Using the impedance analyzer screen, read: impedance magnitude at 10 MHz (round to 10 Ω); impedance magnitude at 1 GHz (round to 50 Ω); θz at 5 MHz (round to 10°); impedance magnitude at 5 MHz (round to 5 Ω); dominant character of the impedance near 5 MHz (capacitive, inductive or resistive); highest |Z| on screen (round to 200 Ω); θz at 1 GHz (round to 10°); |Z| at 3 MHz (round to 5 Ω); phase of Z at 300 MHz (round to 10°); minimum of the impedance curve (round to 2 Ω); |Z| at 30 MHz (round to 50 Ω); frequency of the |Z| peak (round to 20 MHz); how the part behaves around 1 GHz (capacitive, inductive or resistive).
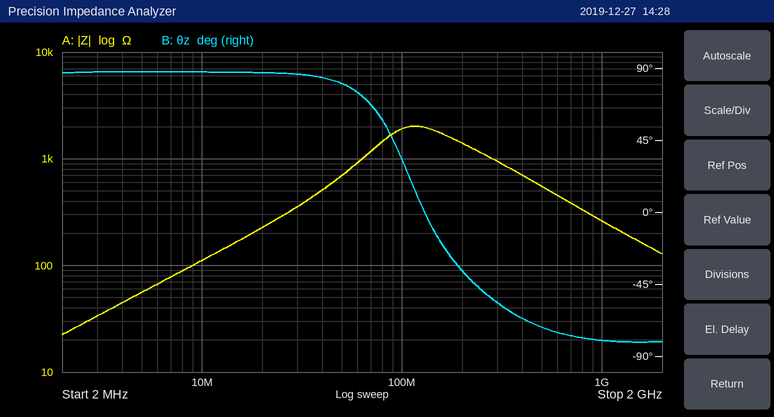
110 Ω
250 Ω
90°
55 Ω
inductive
2.0 kΩ
-80°
35 Ω
-60°
22 Ω
350 Ω
120 MHz
capacitive
